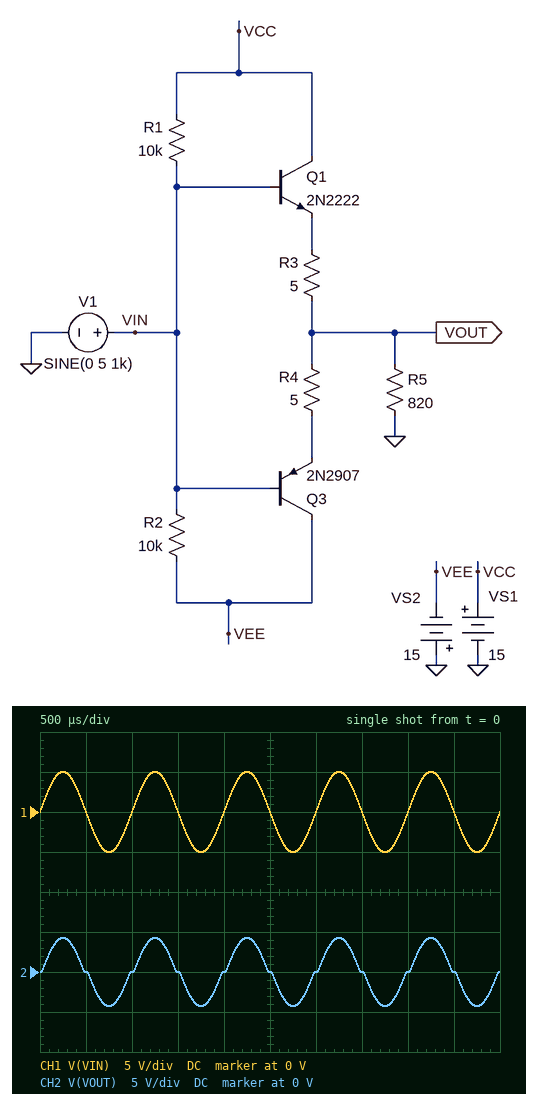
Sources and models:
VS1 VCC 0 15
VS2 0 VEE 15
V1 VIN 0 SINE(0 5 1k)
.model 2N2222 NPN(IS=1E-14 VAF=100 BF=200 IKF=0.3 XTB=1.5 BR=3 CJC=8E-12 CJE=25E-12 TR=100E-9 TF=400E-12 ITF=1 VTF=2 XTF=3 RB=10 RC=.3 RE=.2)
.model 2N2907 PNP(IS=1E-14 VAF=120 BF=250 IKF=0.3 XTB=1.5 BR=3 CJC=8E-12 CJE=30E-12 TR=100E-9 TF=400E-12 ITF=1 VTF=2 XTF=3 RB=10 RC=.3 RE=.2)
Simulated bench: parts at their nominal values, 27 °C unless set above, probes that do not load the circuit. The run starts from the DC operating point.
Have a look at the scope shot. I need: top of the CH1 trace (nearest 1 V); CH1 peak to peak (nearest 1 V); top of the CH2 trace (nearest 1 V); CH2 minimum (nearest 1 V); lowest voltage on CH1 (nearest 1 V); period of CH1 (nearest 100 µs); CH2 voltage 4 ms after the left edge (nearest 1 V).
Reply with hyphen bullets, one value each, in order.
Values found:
- 5 V
- 10 V
- 4 V
- -4 V
- -5 V
- 1.0 ms
- 0 V
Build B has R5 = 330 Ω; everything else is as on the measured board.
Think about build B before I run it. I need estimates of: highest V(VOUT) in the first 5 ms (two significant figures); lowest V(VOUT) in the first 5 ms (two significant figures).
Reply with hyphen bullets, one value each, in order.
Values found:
- 4.2 V
- -4.2 V
